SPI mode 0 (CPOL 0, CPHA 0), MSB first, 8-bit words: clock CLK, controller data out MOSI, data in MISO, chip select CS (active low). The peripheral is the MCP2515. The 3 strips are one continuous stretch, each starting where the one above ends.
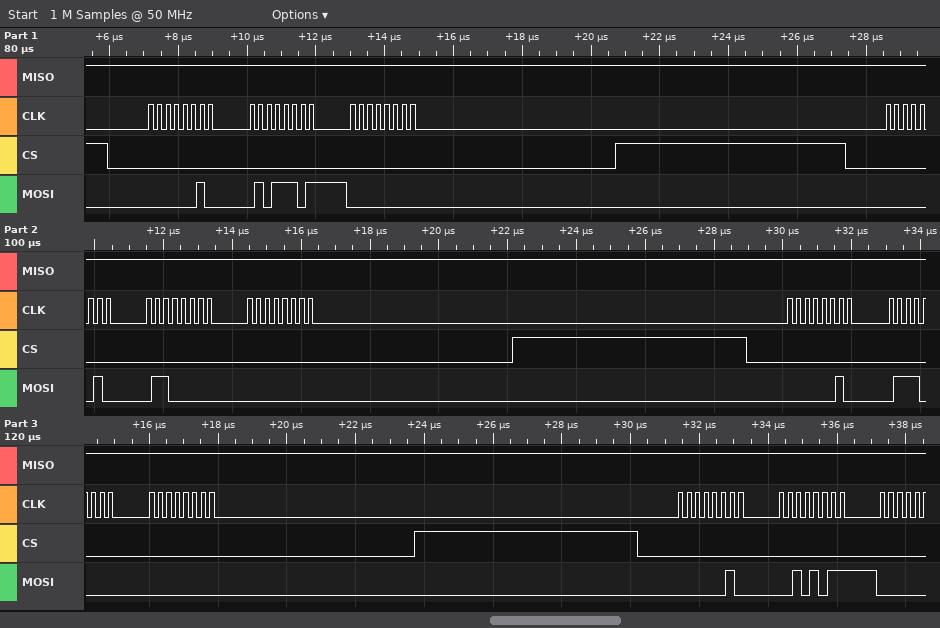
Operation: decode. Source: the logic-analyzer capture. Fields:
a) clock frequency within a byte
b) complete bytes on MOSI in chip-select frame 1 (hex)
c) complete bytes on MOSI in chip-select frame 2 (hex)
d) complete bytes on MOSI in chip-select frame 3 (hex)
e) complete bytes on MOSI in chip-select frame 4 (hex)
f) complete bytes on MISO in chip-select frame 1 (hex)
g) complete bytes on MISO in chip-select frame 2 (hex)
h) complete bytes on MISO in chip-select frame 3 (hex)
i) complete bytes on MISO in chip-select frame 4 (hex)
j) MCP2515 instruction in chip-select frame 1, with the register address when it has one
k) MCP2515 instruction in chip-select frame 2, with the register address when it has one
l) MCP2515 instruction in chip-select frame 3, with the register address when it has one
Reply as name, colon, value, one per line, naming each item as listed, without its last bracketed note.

clock frequency within a byte: 4 MHz
complete bytes on MOSI in chip-select frame 1: 02 5D 00
complete bytes on MOSI in chip-select frame 2: 02 60 00
complete bytes on MOSI in chip-select frame 3: 02 70 00
complete bytes on MOSI in chip-select frame 4: 02 2B
complete bytes on MISO in chip-select frame 1: FF FF FF
complete bytes on MISO in chip-select frame 2: FF FF FF
complete bytes on MISO in chip-select frame 3: FF FF FF
complete bytes on MISO in chip-select frame 4: FF FF
MCP2515 instruction in chip-select frame 1, with the register address when it has one: WRITE 0x5D
MCP2515 instruction in chip-select frame 2, with the register address when it has one: WRITE 0x60
MCP2515 instruction in chip-select frame 3, with the register address when it has one: WRITE 0x70
